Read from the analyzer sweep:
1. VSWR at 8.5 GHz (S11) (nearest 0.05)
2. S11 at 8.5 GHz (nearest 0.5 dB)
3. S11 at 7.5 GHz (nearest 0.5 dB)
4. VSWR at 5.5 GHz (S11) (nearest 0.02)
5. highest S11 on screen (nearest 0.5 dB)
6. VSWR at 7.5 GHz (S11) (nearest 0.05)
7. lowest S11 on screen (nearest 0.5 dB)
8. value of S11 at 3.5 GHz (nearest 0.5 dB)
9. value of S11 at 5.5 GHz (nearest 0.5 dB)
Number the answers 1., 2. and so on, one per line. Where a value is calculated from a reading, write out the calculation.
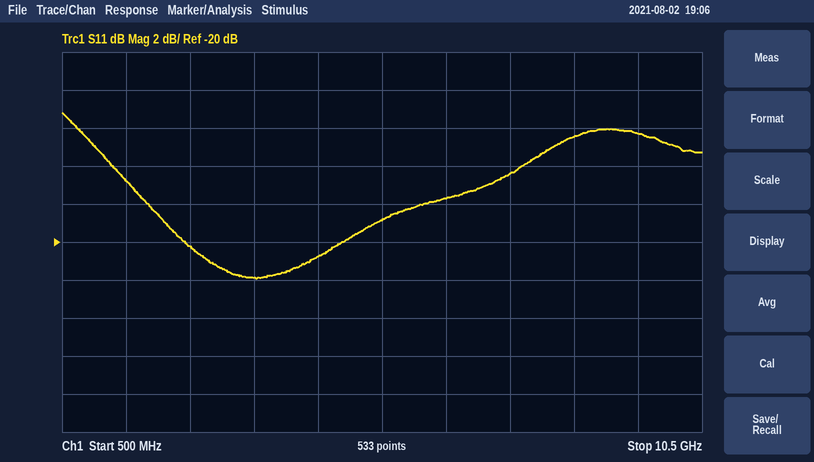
1. |Γ| = 10^(-14.5/20) = 0.1884; VSWR = (1 + 0.1884)/(1 − 0.1884) ≈ 1.46, so 1.45 to the nearest 0.05
2. -14.5 dB
3. -16.5 dB
4. |Γ| = 10^(-19/20) = 0.1122; VSWR = (1 + 0.1122)/(1 − 0.1122) ≈ 1.25, so 1.26 to the nearest 0.02
5. -13.0 dB
6. |Γ| = 10^(-16.5/20) = 0.1496; VSWR = (1 + 0.1496)/(1 − 0.1496) ≈ 1.35
7. -22.0 dB
8. -22.0 dB
9. -19.0 dB
